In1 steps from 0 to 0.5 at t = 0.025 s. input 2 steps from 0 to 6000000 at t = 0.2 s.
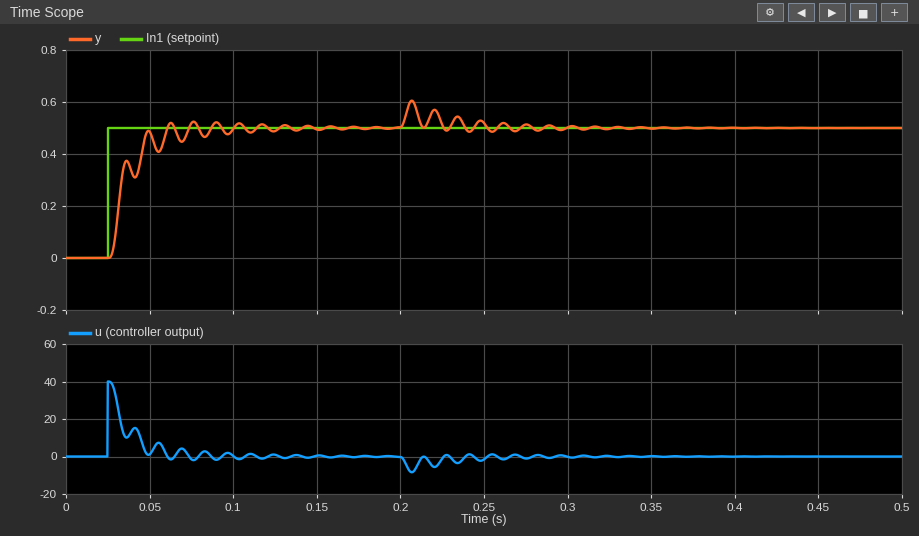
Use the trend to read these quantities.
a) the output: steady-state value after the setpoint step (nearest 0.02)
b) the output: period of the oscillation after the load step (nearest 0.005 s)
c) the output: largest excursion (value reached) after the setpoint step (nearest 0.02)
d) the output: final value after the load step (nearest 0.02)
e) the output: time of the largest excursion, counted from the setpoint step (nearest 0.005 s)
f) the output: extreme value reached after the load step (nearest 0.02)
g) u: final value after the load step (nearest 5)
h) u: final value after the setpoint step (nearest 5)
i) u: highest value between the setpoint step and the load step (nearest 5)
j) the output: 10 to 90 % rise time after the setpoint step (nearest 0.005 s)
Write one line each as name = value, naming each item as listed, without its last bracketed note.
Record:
the output: steady-state value after the setpoint step = 0.50
the output: period of the oscillation after the load step = 0.015 s
the output: largest excursion (value reached) after the setpoint step = 0.52
the output: final value after the load step = 0.50
the output: time of the largest excursion, counted from the setpoint step = 0.050 s
the output: extreme value reached after the load step = 0.60
u: final value after the load step = 0
u: final value after the setpoint step = 0
u: highest value between the setpoint step and the load step = 40
the output: 10 to 90 % rise time after the setpoint step = 0.020 s
